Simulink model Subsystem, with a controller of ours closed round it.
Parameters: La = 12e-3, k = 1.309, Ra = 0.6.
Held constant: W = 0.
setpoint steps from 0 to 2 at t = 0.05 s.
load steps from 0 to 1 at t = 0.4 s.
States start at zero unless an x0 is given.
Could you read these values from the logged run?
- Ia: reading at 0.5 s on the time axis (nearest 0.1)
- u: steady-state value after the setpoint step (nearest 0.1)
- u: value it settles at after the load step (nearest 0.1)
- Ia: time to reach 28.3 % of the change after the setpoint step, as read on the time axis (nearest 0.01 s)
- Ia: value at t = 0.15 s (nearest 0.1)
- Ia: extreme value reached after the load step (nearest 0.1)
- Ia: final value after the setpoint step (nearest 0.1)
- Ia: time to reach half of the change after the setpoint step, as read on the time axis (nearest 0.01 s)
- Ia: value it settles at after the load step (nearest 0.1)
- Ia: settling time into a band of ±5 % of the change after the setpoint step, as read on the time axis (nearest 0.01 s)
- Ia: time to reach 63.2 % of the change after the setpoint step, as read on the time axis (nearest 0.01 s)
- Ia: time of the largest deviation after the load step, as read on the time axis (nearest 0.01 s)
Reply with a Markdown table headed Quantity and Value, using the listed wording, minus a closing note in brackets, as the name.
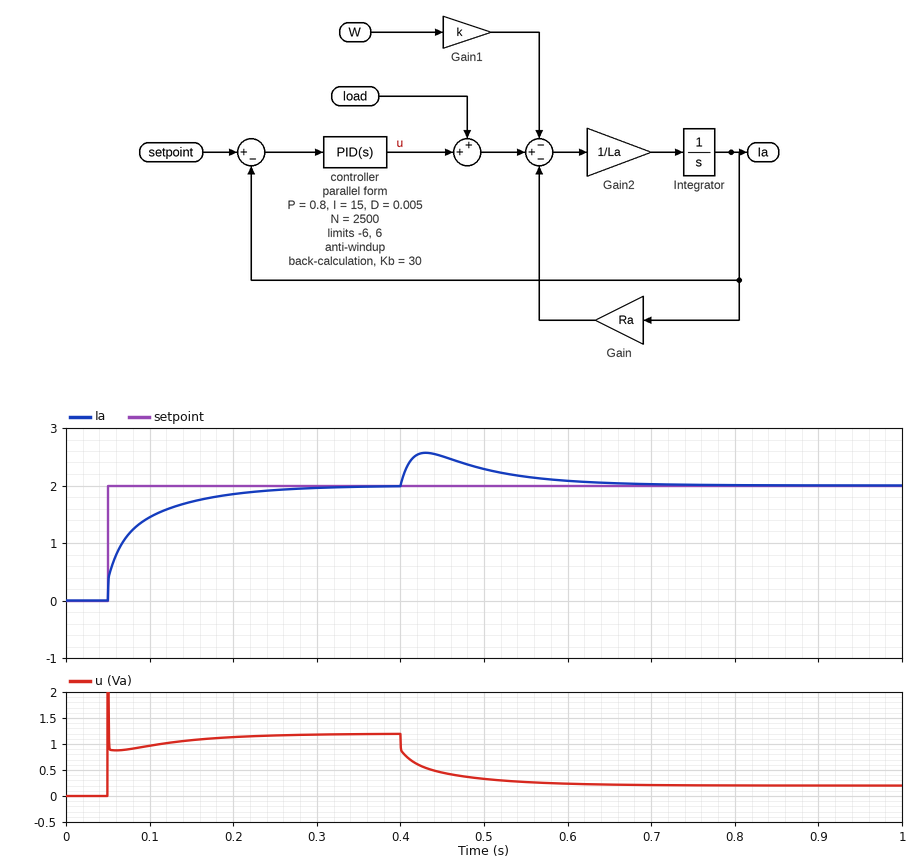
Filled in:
| Quantity | Value |
|---|---|
| Ia: reading at 0.5 s on the time axis | 2.3 |
| u: steady-state value after the setpoint step | 1.2 |
| u: value it settles at after the load step | 0.2 |
| Ia: time to reach 28.3 % of the change after the setpoint step, as read on the time axis | 0.05 s |
| Ia: value at t = 0.15 s | 1.7 |
| Ia: extreme value reached after the load step | 2.6 |
| Ia: final value after the setpoint step | 2.0 |
| Ia: time to reach half of the change after the setpoint step, as read on the time axis | 0.07 s |
| Ia: value it settles at after the load step | 2.0 |
| Ia: settling time into a band of ±5 % of the change after the setpoint step, as read on the time axis | 0.23 s |
| Ia: time to reach 63.2 % of the change after the setpoint step, as read on the time axis | 0.08 s |
| Ia: time of the largest deviation after the load step, as read on the time axis | 0.43 s |
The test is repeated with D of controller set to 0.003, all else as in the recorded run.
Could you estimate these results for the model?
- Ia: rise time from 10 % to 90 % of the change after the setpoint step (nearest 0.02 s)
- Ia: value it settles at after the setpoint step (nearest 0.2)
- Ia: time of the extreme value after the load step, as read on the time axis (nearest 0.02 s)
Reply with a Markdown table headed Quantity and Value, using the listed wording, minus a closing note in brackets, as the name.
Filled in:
| Quantity | Value |
|---|---|
| Ia: rise time from 10 % to 90 % of the change after the setpoint step | 0.12 s |
| Ia: value it settles at after the setpoint step | 2.0 |
| Ia: time of the extreme value after the load step, as read on the time axis | 0.42 s |
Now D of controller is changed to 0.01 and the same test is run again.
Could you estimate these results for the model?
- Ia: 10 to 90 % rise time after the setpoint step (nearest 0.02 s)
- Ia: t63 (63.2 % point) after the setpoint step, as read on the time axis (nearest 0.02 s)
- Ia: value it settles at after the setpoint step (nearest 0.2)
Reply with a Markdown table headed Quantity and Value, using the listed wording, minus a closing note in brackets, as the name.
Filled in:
| Quantity | Value |
|---|---|
| Ia: 10 to 90 % rise time after the setpoint step | 0.14 s |
| Ia: t63 (63.2 % point) after the setpoint step, as read on the time axis | 0.10 s |
| Ia: value it settles at after the setpoint step | 2.0 |
